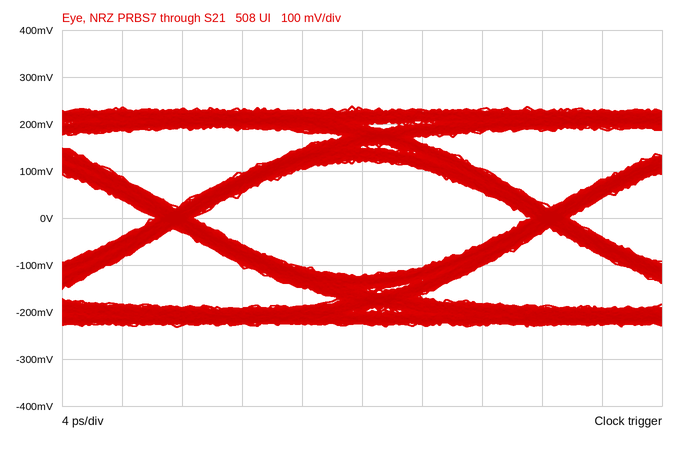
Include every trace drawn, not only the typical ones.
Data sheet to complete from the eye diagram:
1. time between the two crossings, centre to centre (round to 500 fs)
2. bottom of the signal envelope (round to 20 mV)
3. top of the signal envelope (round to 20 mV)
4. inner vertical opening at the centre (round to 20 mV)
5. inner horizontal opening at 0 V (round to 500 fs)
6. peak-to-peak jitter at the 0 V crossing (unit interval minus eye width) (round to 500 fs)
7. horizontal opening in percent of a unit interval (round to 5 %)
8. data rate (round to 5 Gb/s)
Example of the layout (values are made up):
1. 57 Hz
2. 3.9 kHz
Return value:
1. 25.0 ps
2. -240 mV
3. 240 mV
4. 240 mV
5. 22.5 ps
6. 2.5 ps
7. 90 %
8. 40 Gb/s
